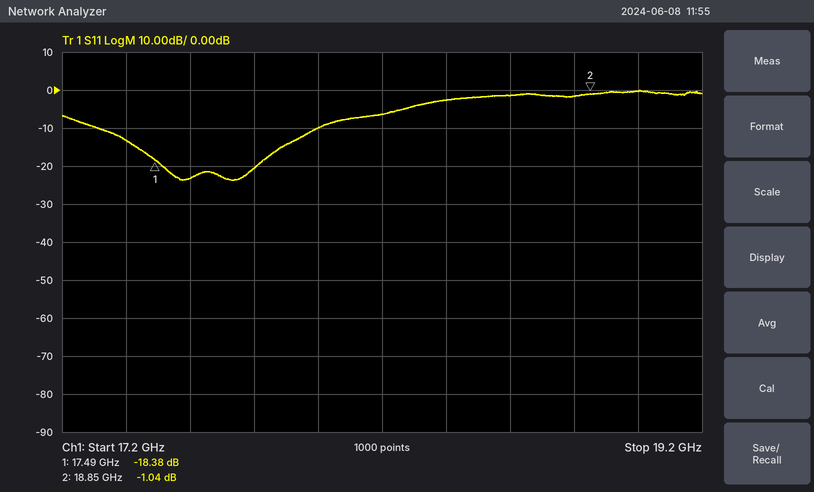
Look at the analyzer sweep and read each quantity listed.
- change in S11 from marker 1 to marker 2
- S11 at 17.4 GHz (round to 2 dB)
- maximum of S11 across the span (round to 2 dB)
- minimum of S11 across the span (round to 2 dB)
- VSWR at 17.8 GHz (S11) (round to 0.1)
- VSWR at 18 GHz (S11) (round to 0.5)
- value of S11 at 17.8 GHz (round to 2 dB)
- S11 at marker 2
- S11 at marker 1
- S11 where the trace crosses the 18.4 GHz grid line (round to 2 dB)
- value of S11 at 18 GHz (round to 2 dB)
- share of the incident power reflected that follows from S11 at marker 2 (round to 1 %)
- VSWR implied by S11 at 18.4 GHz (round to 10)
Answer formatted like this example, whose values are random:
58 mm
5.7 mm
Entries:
17.34 dB
-14 dB
0 dB
-24 dB
1.2
2.0
-20 dB
-1.04 dB
-18.38 dB
-2 dB
-10 dB
79 %
10
